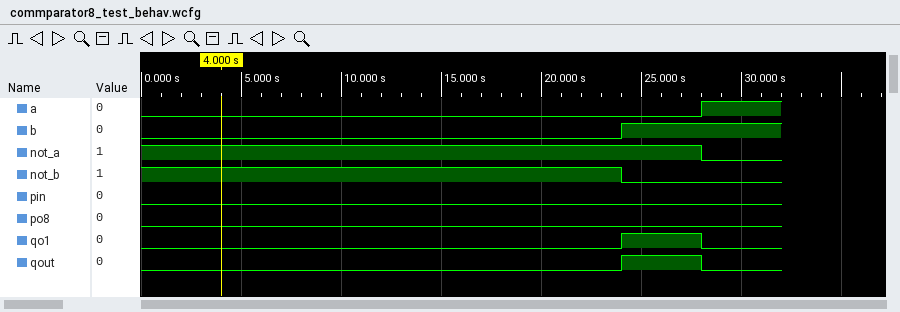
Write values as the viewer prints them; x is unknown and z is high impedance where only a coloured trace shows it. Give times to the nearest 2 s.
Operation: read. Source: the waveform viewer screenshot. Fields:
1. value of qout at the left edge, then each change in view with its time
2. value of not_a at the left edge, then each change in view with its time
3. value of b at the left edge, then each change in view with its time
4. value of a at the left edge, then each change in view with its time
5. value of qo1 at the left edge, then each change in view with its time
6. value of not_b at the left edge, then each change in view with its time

0, 1 at 24 s, 0 at 28 s
1, 0 at 28 s
0, 1 at 24 s
0, 1 at 28 s
0, 1 at 24 s, 0 at 28 s
1, 0 at 24 s
